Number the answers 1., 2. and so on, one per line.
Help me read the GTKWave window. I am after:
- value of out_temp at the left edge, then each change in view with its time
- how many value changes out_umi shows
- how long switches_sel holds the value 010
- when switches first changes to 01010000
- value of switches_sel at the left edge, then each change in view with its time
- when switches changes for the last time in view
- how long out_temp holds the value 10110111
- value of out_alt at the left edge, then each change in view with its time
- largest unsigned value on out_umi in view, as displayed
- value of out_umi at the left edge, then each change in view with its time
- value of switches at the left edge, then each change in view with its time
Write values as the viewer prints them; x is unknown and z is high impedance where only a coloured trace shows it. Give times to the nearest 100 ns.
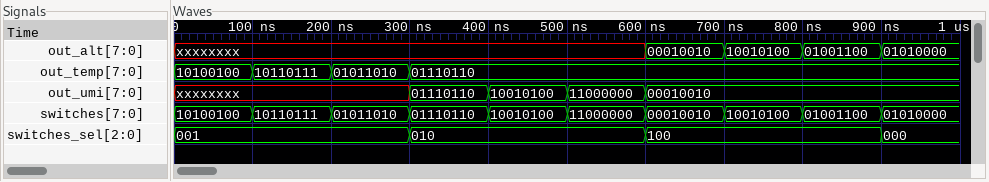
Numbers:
1. 10100100, 10110111 at 100 ns, 01011010 at 200 ns, 01110110 at 300 ns
2. 4
3. 300 ns
4. 900 ns
5. 001, 010 at 300 ns, 100 at 600 ns, 000 at 900 ns
6. 900 ns
7. 100 ns
8. xxxxxxxx, 00010010 at 600 ns, 10010100 at 700 ns, 01001100 at 800 ns, 01010000 at 900 ns
9. 11000000
10. xxxxxxxx, 01110110 at 300 ns, 10010100 at 400 ns, 11000000 at 500 ns, 00010010 at 600 ns
11. 10100100, 10110111 at 100 ns, 01011010 at 200 ns, 01110110 at 300 ns, 10010100 at 400 ns, 11000000 at 500 ns, 00010010 at 600 ns, 10010100 at 700 ns, 01001100 at 800 ns, 01010000 at 900 ns
